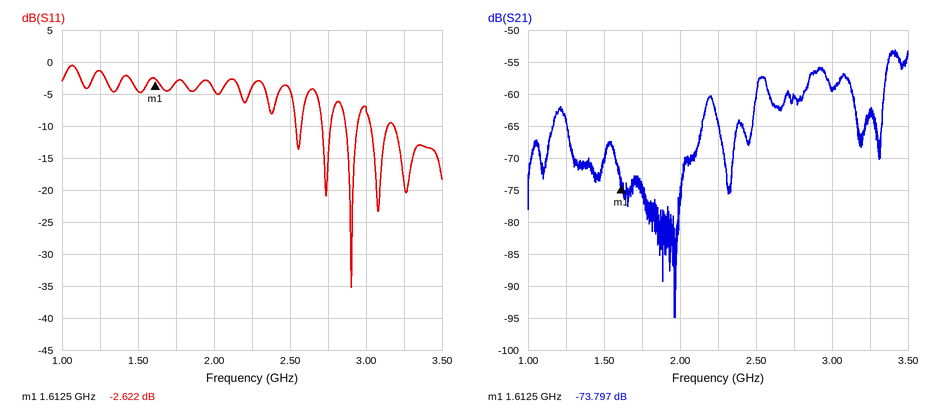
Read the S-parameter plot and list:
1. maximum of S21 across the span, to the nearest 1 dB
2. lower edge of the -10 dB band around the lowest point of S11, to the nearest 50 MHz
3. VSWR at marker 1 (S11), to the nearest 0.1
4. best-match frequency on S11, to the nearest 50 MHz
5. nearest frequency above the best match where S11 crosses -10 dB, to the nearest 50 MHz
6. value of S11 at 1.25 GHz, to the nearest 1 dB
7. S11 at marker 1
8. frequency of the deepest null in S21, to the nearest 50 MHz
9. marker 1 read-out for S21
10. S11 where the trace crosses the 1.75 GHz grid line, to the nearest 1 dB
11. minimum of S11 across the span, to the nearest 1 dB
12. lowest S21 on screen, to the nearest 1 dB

-53 dB
2.85 GHz
6.7
2.90 GHz
2.95 GHz
-1 dB
-2.622 dB
1.95 GHz
-73.797 dB
-3 dB
-35 dB
-95 dB
